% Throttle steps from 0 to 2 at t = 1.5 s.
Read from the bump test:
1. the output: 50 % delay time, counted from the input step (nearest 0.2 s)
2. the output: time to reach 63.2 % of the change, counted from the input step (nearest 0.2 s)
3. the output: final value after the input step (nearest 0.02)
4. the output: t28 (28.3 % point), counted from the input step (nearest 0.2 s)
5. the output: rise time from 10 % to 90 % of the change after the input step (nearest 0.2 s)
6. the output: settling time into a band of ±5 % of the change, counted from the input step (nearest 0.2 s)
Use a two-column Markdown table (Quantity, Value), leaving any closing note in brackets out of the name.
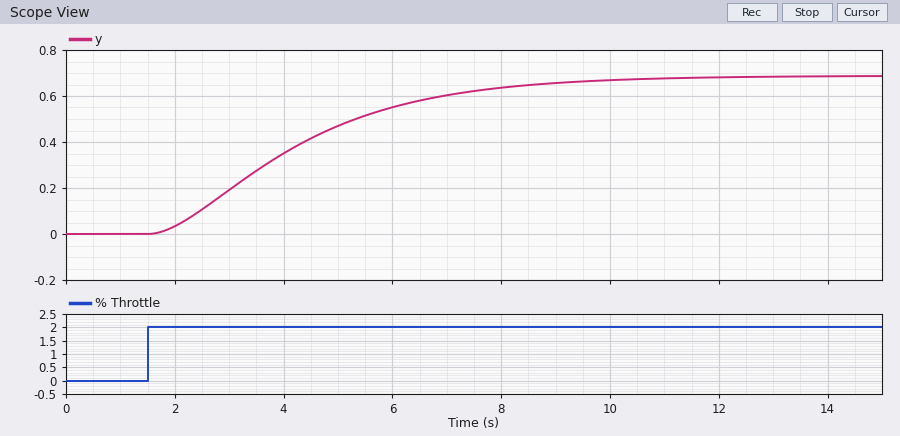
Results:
| Quantity | Value |
|---|---|
| the output: 50 % delay time, counted from the input step | 2.4 s |
| the output: time to reach 63.2 % of the change, counted from the input step | 3.2 s |
| the output: final value after the input step | 0.68 |
| the output: t28 (28.3 % point), counted from the input step | 1.6 s |
| the output: rise time from 10 % to 90 % of the change after the input step | 5.2 s |
| the output: settling time into a band of ±5 % of the change, counted from the input step | 7.4 s |
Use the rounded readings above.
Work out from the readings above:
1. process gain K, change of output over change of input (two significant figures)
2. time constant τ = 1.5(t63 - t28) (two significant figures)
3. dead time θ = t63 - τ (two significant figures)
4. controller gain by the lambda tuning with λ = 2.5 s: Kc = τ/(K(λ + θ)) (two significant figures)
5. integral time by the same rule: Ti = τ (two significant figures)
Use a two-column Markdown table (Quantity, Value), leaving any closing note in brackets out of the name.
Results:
| Quantity | Value |
|---|---|
| process gain K, change of output over change of input | 0.34 |
| time constant τ = 1.5(t63 - t28) | 2.4 s |
| dead time θ = t63 - τ | 0.80 s |
| controller gain by the lambda tuning with λ = 2.5 s: Kc = τ/(K(λ + θ)) | 2.1 |
| integral time by the same rule: Ti = τ | 2.4 s |
